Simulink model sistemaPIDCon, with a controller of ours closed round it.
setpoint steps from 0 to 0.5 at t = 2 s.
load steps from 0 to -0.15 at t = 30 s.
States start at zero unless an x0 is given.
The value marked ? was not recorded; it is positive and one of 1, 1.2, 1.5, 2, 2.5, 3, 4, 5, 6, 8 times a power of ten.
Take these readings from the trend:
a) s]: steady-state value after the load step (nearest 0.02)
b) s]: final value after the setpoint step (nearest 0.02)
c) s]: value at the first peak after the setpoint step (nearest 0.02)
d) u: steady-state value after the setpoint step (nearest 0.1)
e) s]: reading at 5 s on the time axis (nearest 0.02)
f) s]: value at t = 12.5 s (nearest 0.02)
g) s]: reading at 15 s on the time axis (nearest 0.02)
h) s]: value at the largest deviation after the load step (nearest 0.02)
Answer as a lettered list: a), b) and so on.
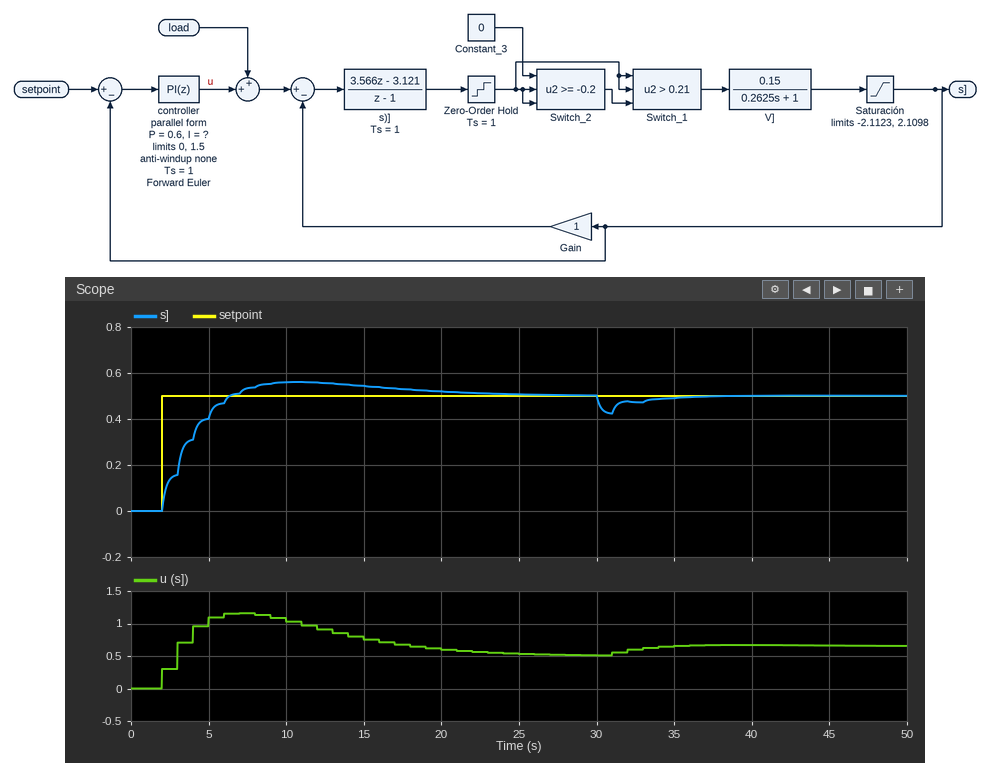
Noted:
a) 0.50
b) 0.50
c) 0.56
d) 0.5
e) 0.40
f) 0.56
g) 0.54
h) 0.42
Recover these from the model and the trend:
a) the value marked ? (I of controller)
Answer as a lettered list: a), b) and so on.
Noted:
a) 1
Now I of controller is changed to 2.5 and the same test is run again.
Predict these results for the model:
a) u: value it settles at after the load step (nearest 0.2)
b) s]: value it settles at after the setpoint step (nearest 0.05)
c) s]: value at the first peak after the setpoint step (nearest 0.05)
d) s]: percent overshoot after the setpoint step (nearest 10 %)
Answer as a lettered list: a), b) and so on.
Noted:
a) 0.6
b) 0.50
c) 0.70
d) 40 %
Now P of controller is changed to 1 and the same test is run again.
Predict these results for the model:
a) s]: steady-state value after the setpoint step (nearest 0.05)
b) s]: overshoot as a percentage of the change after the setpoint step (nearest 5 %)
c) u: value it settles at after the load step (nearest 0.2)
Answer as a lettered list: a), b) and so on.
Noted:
a) 0.50
b) 10 %
c) 0.6
